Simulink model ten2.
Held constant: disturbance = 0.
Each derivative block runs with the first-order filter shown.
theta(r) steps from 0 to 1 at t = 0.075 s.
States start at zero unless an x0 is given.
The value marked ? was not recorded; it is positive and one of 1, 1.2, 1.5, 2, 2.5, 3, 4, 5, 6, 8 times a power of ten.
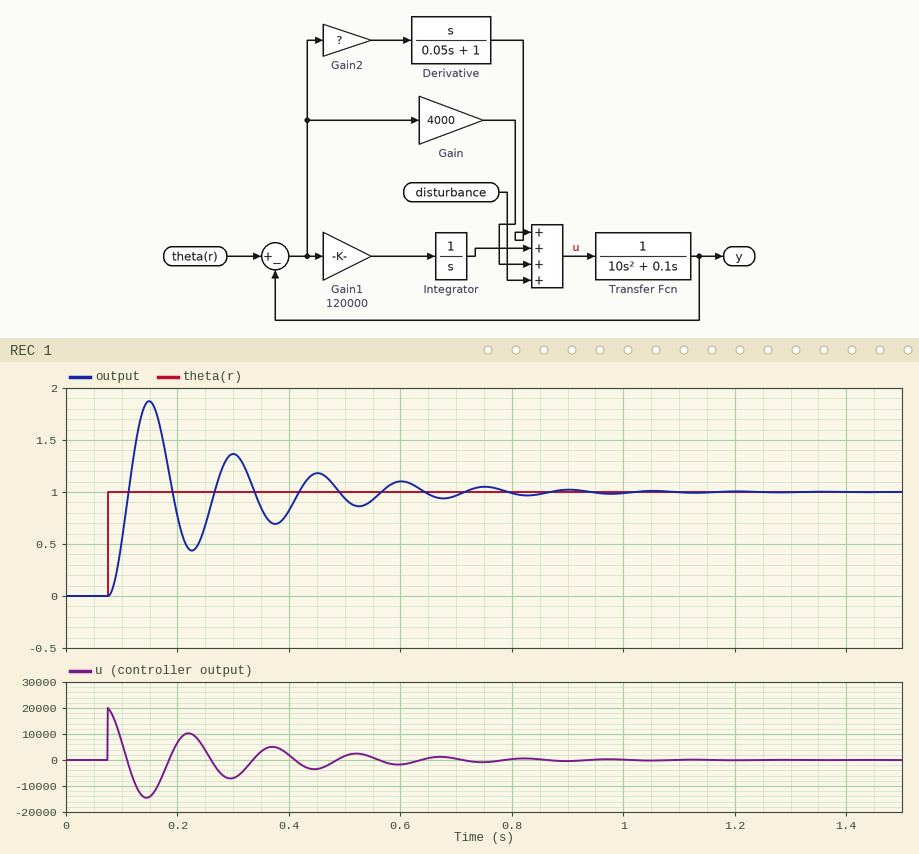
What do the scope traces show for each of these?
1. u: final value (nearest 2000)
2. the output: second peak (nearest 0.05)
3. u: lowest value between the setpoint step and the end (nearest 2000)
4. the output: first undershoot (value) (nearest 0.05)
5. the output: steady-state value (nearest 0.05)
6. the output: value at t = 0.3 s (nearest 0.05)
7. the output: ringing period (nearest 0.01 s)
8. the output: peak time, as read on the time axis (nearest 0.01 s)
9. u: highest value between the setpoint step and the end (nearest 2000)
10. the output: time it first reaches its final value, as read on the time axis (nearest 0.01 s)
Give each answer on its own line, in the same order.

0
1.35
-14000
0.45
1.00
1.35
0.15 s
0.15 s
20000
0.11 s
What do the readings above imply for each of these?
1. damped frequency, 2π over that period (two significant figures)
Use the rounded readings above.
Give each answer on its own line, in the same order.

42 rad/s
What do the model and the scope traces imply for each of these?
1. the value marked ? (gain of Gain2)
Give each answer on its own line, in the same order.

800
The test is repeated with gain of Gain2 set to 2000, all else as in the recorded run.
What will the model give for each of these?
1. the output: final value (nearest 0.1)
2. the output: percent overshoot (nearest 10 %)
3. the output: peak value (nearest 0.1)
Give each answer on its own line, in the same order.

1.0
70 %
1.7
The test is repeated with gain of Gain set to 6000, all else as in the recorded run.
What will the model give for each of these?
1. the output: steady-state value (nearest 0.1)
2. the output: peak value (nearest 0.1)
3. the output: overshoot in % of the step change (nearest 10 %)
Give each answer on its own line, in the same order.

1.0
1.9
90 %
